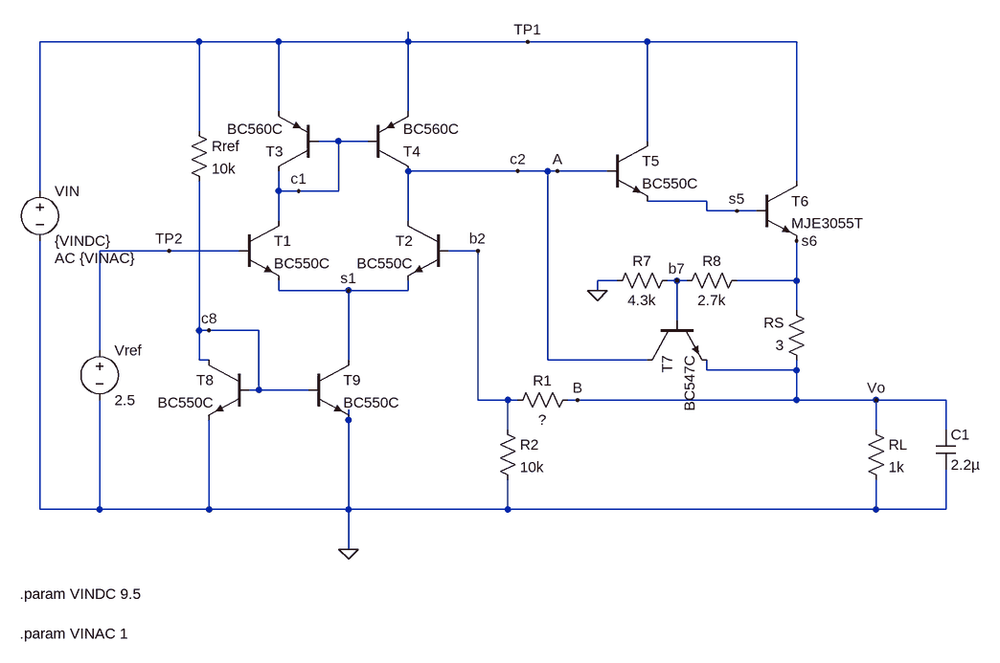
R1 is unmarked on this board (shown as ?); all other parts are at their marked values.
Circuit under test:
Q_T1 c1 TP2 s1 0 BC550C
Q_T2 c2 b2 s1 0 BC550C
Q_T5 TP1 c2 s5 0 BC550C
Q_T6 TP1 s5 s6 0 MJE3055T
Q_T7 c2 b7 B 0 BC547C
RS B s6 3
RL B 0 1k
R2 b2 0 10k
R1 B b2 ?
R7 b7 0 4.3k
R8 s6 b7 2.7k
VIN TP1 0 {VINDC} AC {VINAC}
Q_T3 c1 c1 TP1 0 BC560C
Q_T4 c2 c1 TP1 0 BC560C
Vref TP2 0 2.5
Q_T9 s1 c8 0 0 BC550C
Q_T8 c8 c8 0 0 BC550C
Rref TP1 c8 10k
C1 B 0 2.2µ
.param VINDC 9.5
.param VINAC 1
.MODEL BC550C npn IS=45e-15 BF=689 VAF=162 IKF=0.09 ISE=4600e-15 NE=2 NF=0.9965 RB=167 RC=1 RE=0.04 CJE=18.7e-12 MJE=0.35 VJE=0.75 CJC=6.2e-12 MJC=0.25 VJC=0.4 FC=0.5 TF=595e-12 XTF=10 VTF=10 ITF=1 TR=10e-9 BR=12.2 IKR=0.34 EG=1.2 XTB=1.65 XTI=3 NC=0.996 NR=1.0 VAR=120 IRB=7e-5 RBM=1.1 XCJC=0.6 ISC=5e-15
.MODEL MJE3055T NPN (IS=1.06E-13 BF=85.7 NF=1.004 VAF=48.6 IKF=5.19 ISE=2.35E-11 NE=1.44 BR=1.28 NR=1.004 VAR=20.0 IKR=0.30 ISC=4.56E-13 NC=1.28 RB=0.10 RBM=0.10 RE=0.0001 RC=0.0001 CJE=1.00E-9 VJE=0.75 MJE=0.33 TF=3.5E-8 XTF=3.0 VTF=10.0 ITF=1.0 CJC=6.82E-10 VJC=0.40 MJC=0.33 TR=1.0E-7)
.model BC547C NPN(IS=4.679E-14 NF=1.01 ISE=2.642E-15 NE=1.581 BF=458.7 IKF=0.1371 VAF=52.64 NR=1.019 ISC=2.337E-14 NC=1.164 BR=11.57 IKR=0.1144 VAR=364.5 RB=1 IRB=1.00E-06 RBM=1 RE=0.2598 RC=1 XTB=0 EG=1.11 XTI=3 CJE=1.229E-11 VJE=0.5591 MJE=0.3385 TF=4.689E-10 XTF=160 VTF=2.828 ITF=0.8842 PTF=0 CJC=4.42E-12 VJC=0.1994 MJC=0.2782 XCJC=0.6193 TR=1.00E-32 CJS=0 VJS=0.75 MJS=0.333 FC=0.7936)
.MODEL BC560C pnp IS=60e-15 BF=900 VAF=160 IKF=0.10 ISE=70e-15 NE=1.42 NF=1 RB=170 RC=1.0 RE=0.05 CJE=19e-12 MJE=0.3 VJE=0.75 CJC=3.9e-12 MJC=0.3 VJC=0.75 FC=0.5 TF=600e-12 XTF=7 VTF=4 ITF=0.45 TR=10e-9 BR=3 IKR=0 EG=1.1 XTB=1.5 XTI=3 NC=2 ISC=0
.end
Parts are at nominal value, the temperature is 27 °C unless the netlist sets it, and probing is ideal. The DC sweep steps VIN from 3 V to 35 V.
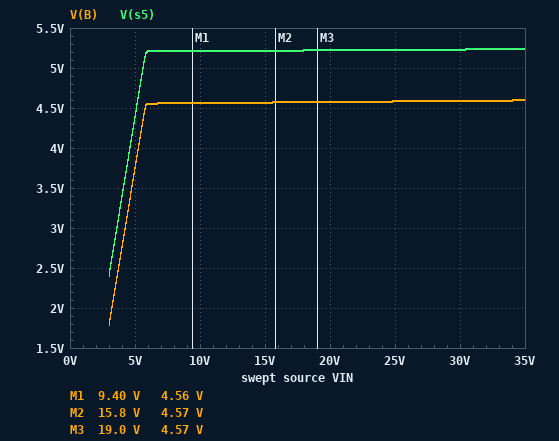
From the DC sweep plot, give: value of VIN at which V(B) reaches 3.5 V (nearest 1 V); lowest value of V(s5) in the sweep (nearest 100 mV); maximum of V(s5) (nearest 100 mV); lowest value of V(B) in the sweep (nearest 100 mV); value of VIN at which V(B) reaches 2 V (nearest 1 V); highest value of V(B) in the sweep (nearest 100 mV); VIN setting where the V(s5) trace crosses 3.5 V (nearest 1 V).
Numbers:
5 V
2.4 V
5.2 V
1.8 V
3 V
4.6 V
4 V
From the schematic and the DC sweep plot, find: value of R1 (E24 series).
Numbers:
8.2 kΩ
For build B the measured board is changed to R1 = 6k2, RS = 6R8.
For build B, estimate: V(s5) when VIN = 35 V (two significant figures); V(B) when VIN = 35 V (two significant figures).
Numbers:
4.7 V
4.1 V
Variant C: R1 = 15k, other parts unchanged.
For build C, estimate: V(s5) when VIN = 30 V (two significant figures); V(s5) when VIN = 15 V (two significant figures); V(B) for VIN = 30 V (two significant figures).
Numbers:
7.0 V
6.9 V
6.3 V
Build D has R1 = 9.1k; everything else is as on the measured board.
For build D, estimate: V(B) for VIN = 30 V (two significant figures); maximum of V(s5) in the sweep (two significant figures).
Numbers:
4.8 V
5.5 V
